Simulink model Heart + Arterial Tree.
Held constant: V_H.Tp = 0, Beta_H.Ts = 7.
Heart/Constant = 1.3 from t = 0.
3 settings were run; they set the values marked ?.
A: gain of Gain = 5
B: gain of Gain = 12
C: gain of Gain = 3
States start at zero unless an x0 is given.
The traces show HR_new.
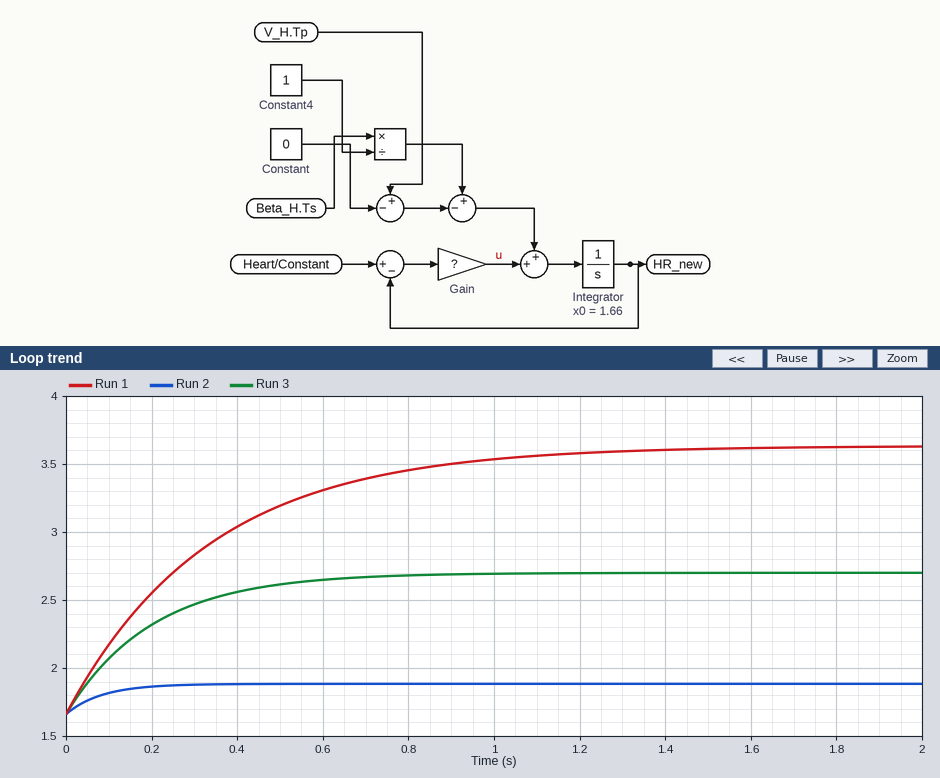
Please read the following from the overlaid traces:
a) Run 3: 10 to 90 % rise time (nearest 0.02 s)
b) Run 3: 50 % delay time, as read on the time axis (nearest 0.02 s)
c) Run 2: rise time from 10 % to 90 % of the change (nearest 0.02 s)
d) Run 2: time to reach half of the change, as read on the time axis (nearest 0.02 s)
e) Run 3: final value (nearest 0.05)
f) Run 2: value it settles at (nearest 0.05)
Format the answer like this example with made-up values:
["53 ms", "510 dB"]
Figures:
["0.44 s", "0.14 s", "0.18 s", "0.06 s", "2.70", "1.90"]
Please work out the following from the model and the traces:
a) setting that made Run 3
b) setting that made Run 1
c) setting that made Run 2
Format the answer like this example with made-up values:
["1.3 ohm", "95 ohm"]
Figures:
["A", "C", "B"]
